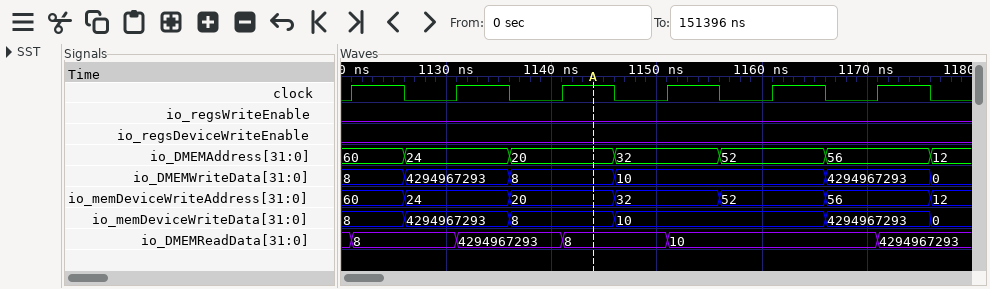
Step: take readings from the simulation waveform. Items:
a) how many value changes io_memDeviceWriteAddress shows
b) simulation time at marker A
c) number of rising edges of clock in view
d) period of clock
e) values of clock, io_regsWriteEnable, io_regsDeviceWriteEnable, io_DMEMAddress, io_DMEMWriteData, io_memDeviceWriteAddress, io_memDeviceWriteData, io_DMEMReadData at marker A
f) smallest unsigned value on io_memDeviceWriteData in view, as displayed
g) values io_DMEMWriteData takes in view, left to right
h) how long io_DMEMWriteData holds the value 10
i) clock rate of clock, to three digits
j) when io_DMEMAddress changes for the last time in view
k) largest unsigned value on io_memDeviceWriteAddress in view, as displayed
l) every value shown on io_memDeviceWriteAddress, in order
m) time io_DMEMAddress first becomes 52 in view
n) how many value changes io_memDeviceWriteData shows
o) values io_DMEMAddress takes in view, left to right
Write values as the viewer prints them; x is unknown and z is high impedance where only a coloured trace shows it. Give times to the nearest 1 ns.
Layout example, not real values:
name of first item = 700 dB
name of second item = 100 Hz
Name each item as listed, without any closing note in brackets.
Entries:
how many value changes io_memDeviceWriteAddress shows = 6
simulation time at marker A = 1144 ns
number of rising edges of clock in view = 6
period of clock = 10 ns
values of clock, io_regsWriteEnable, io_regsDeviceWriteEnable, io_DMEMAddress, io_DMEMWriteData, io_memDeviceWriteAddress, io_memDeviceWriteData, io_DMEMReadData at marker A = clock=1, io_regsWriteEnable=0, io_regsDeviceWriteEnable=0, io_DMEMAddress=20, io_DMEMWriteData=8, io_memDeviceWriteAddress=20, io_memDeviceWriteData=8, io_DMEMReadData=8
smallest unsigned value on io_memDeviceWriteData in view, as displayed = 0
values io_DMEMWriteData takes in view, left to right = 8, 4294967293, 8, 10, 4294967293, 0
how long io_DMEMWriteData holds the value 10 = 20 ns
clock rate of clock, to three digits = 100 MHz
when io_DMEMAddress changes for the last time in view = 1176 ns
largest unsigned value on io_memDeviceWriteAddress in view, as displayed = 60
every value shown on io_memDeviceWriteAddress, in order = 60, 24, 20, 32, 52, 56, 12
time io_DMEMAddress first becomes 52 in view = 1156 ns
how many value changes io_memDeviceWriteData shows = 5
values io_DMEMAddress takes in view, left to right = 60, 24, 20, 32, 52, 56, 12
